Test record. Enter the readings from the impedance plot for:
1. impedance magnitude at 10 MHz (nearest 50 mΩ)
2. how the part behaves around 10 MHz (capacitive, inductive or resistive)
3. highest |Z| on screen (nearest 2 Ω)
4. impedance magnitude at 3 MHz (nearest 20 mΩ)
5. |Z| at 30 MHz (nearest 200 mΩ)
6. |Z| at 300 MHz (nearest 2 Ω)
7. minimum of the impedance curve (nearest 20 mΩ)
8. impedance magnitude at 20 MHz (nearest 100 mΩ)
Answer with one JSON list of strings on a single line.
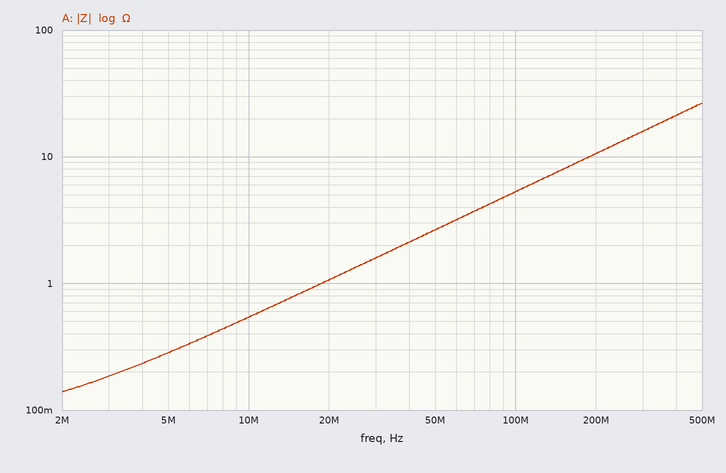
["550 mΩ", "inductive", "26 Ω", "180 mΩ", "1.6 Ω", "16 Ω", "140 mΩ", "1.1 Ω"]
